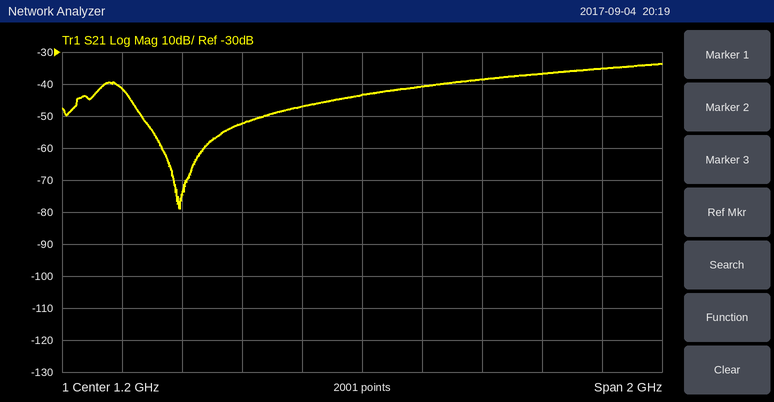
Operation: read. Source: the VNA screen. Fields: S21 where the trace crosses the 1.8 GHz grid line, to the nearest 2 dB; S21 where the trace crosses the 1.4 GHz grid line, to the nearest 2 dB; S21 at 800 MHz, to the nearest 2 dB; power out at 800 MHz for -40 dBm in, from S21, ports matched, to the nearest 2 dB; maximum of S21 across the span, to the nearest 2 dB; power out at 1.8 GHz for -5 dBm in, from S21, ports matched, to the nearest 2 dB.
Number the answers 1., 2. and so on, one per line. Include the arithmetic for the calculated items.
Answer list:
1. -36 dB
2. -40 dB
3. -52 dB
4. -40 dBm + (-52 dB) = -92 dBm
5. -34 dB
6. -5 dBm + (-36 dB) = -42 dBm
